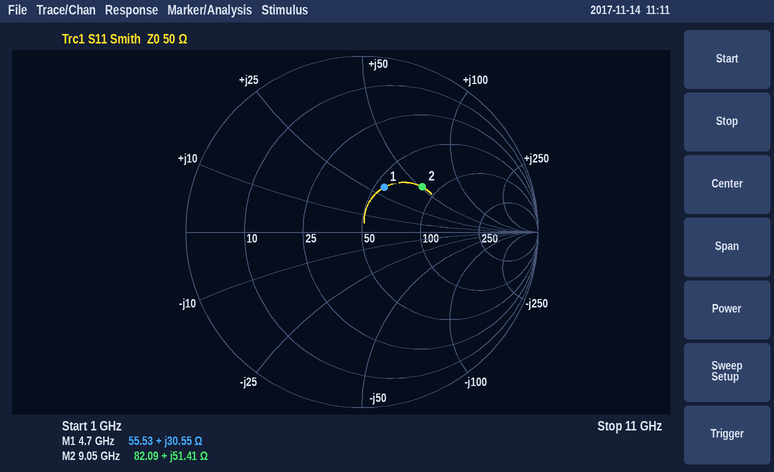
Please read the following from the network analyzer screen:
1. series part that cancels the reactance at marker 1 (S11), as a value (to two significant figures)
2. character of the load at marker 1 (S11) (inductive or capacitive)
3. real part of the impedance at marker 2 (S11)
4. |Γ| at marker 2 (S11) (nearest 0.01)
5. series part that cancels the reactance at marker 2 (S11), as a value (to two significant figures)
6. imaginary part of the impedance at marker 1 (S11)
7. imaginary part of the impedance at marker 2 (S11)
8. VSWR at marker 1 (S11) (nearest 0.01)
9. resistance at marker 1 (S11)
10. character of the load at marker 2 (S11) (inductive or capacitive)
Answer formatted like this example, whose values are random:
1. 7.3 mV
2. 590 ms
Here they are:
1. 1.1 pF
2. inductive
3. 82.09 Ω
4. 0.43
5. 340 fF
6. +30.55 Ω
7. +51.41 Ω
8. 1.79
9. 55.53 Ω
10. inductive
